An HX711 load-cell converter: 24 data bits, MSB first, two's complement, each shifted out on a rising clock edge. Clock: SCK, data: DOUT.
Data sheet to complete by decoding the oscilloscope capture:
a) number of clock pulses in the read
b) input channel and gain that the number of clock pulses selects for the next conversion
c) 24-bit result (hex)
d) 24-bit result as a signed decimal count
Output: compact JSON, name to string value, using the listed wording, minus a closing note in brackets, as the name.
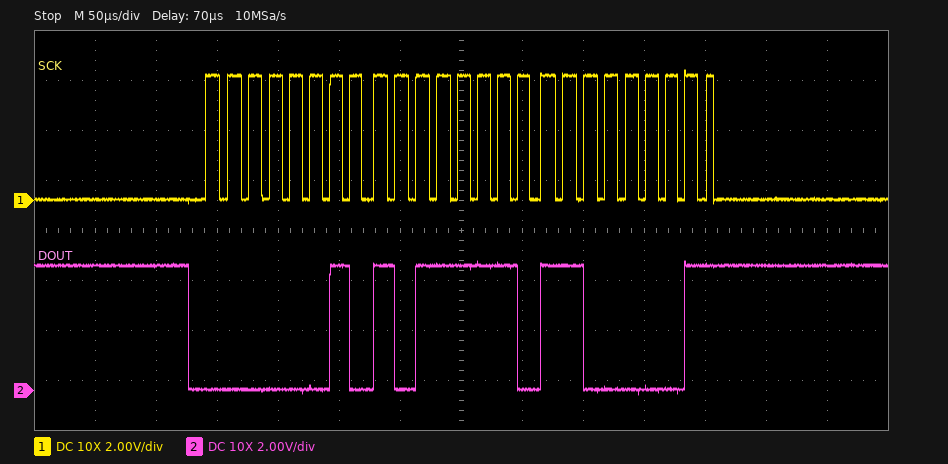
{"number of clock pulses in the read": "25", "input channel and gain that the number of clock pulses selects for the next conversion": "channel A, gain 128", "24-bit result": "0x02BEC1", "24-bit result as a signed decimal count": "179905"}
